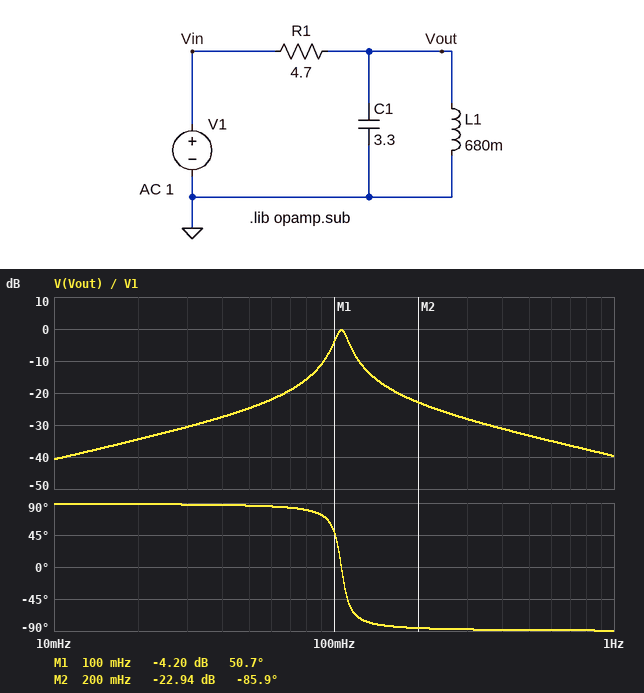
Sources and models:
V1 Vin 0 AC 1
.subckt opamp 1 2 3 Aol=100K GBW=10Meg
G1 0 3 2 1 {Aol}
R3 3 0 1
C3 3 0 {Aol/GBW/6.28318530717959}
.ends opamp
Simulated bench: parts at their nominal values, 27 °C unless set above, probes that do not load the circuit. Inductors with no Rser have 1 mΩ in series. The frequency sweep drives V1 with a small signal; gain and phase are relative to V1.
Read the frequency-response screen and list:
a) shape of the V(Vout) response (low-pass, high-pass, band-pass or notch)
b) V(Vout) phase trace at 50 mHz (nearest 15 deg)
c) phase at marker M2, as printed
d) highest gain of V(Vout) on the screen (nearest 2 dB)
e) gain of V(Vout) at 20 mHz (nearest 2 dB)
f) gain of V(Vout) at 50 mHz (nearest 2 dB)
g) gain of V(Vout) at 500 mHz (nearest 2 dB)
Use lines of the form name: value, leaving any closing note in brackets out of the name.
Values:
shape of the V(Vout) response: band-pass
V(Vout) phase trace at 50 mHz: 90 deg
phase at marker M2, as printed: -85.9 deg
highest gain of V(Vout) on the screen: 0 dB
gain of V(Vout) at 20 mHz: -34 dB
gain of V(Vout) at 50 mHz: -24 dB
gain of V(Vout) at 500 mHz: -34 dB
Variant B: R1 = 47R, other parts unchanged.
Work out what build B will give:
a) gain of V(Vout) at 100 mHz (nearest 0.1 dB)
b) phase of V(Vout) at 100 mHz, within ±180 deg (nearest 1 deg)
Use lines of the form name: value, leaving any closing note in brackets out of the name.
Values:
gain of V(Vout) at 100 mHz: -22.0 dB
phase of V(Vout) at 100 mHz, within ±180 deg: 84 deg
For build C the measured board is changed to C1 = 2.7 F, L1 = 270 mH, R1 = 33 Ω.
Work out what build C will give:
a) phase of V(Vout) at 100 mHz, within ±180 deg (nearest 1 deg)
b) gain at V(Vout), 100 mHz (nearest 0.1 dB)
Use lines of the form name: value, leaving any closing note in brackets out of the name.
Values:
phase of V(Vout) at 100 mHz, within ±180 deg: 89 deg
gain at V(Vout), 100 mHz: -42.8 dB
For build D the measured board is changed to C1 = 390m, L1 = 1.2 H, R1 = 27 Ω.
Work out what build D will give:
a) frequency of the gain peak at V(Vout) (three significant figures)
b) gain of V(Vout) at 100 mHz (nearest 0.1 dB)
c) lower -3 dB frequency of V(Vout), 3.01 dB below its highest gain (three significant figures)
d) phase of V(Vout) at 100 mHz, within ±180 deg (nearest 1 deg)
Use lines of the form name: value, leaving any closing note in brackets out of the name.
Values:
frequency of the gain peak at V(Vout): 233 mHz
gain of V(Vout) at 100 mHz: -29.3 dB
lower -3 dB frequency of V(Vout), 3.01 dB below its highest gain: 225 mHz
phase of V(Vout) at 100 mHz, within ±180 deg: 88 deg
